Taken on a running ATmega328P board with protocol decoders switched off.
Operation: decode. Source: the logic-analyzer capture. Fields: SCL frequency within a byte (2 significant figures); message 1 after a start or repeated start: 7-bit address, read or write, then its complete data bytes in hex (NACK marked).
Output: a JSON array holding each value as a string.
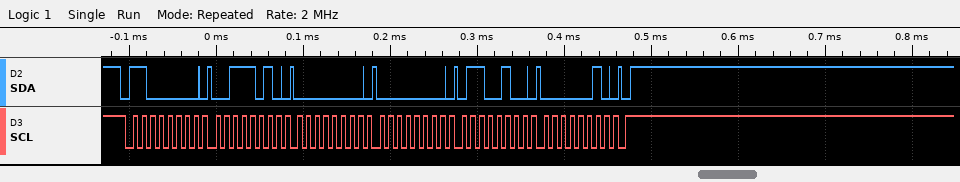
["100 kHz", "0x60 write: 3A 00 00 64 02"]
